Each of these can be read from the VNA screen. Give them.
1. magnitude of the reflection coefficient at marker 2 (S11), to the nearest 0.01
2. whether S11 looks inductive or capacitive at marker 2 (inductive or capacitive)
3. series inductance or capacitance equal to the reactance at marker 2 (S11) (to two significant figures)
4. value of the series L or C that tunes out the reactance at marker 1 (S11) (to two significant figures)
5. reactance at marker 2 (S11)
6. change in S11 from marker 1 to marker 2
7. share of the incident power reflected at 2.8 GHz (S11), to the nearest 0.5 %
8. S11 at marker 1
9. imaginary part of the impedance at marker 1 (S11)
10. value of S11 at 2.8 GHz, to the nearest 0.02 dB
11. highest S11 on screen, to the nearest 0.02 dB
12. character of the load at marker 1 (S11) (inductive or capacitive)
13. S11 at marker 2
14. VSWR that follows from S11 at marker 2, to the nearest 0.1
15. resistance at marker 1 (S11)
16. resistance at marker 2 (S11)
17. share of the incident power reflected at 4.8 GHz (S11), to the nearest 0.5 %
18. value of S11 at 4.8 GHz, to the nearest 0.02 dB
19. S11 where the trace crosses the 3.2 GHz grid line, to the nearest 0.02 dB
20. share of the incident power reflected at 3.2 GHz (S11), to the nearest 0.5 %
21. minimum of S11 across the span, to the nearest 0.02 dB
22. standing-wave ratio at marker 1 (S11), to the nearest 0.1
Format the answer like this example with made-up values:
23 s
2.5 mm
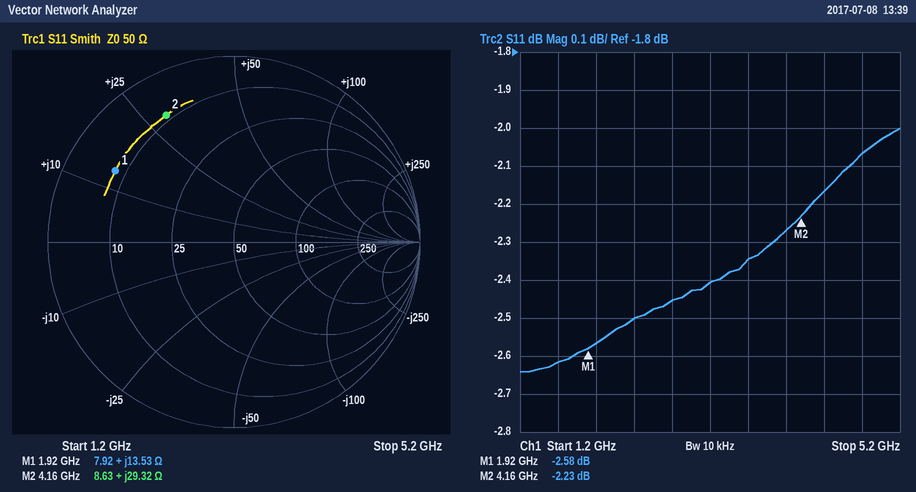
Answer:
0.77
inductive
1.1 nH
6.1 pF
+29.32 Ω
0.35 dB
57.0 %
-2.58 dB
+13.53 Ω
-2.46 dB
-2.00 dB
inductive
-2.23 dB
7.8
7.92 Ω
8.63 Ω
62.0 %
-2.06 dB
-2.40 dB
57.5 %
-2.64 dB
6.8
